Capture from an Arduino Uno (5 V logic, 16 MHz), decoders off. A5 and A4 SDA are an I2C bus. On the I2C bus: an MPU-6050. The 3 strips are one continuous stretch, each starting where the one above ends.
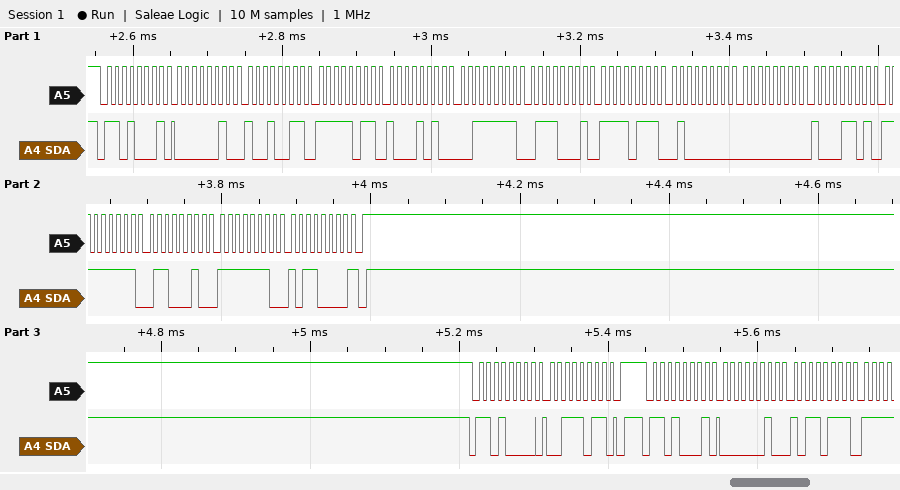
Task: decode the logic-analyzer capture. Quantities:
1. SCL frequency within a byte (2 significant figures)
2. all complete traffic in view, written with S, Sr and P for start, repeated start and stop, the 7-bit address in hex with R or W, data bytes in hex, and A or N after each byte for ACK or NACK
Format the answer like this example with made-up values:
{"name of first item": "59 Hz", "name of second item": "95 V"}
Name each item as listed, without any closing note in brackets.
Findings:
{"SCL frequency within a byte": "100 kHz", "all complete traffic in view, written with S, Sr and P for start, repeated start and stop, the 7-bit address in hex with R or W, data bytes in hex, and A or N after each byte for ACK or NACK": "S 68R A 02 A 93 A FB A 8A A 3F A 71 A F7 A 40 A 00 A 8D A FF A 62 A FE A B0 N P S 68W A 3B A P S 68R A 02 A B7 A"}
